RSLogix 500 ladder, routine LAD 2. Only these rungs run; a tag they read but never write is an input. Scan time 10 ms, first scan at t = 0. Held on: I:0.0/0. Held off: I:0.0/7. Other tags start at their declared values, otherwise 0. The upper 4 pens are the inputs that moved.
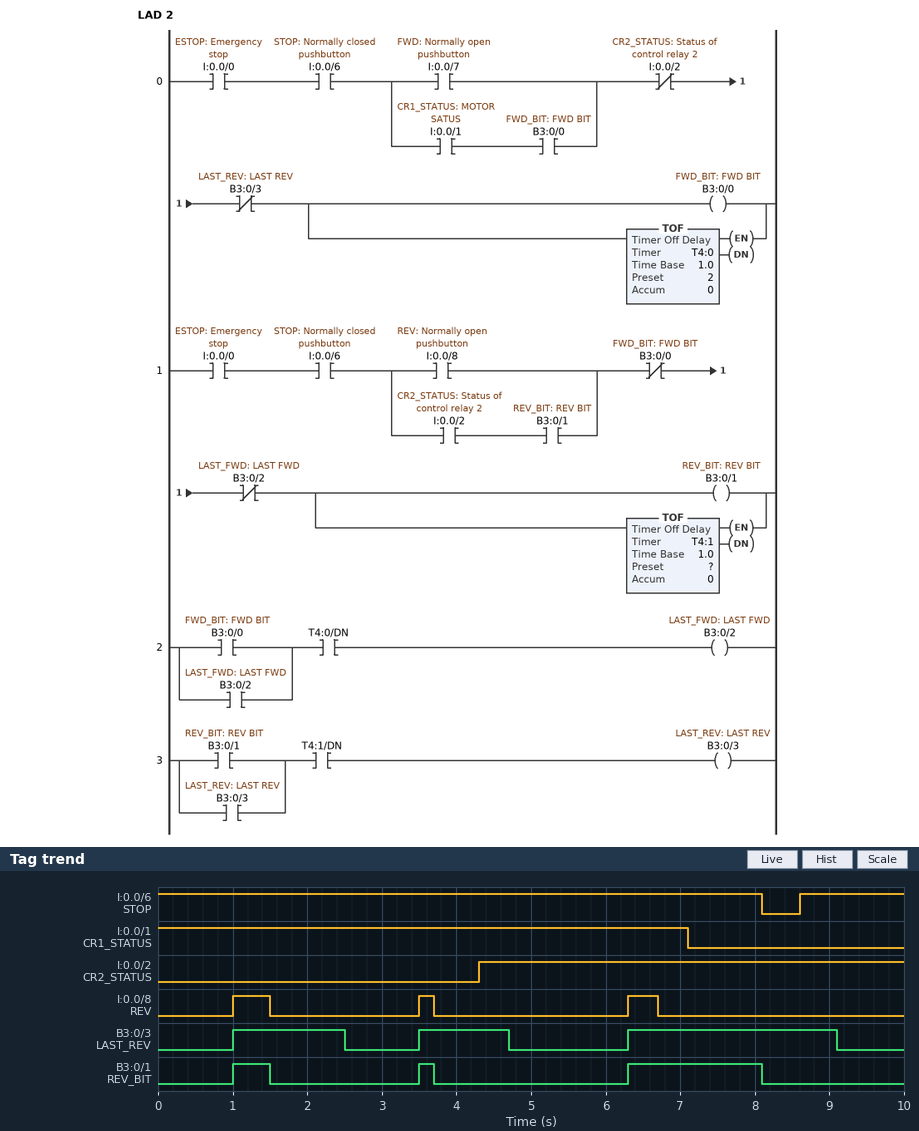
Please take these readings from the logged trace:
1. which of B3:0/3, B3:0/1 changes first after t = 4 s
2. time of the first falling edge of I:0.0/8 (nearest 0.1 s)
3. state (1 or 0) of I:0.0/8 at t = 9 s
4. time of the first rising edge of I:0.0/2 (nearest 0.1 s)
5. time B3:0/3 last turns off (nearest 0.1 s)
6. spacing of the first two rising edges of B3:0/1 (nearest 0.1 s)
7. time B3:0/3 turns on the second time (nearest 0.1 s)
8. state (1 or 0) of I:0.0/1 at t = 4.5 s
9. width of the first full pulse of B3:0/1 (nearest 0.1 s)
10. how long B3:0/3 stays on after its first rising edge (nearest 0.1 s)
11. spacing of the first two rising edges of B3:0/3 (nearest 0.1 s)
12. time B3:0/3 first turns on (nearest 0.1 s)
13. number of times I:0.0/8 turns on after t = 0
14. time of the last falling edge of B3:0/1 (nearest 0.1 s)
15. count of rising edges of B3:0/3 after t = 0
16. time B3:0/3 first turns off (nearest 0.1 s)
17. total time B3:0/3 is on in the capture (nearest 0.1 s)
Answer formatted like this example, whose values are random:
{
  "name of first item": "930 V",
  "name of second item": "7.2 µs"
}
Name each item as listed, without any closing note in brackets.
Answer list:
{
  "which of B3:0/3, B3:0/1 changes first after t = 4 s": "B3:0/3",
  "time of the first falling edge of I:0.0/8": "1.5 s",
  "state (1 or 0) of I:0.0/8 at t = 9 s": "0",
  "time of the first rising edge of I:0.0/2": "4.3 s",
  "time B3:0/3 last turns off": "9.1 s",
  "spacing of the first two rising edges of B3:0/1": "2.5 s",
  "time B3:0/3 turns on the second time": "3.5 s",
  "state (1 or 0) of I:0.0/1 at t = 4.5 s": "1",
  "width of the first full pulse of B3:0/1": "0.5 s",
  "how long B3:0/3 stays on after its first rising edge": "1.5 s",
  "spacing of the first two rising edges of B3:0/3": "2.5 s",
  "time B3:0/3 first turns on": "1.0 s",
  "number of times I:0.0/8 turns on after t = 0": "3",
  "time of the last falling edge of B3:0/1": "8.1 s",
  "count of rising edges of B3:0/3 after t = 0": "3",
  "time B3:0/3 first turns off": "2.5 s",
  "total time B3:0/3 is on in the capture": "5.5 s"
}
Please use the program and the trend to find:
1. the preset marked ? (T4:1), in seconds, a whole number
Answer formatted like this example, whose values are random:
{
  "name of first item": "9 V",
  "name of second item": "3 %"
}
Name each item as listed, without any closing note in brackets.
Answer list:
{
  "the preset marked ? (T4:1), in seconds, a whole number": "1 s"
}
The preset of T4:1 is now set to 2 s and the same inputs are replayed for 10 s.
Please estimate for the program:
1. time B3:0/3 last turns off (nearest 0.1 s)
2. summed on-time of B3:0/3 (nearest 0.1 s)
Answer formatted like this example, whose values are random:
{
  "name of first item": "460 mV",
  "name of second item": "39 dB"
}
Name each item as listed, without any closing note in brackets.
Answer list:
{
  "time B3:0/3 last turns off": "5.7 s",
  "summed on-time of B3:0/3": "8.4 s"
}
